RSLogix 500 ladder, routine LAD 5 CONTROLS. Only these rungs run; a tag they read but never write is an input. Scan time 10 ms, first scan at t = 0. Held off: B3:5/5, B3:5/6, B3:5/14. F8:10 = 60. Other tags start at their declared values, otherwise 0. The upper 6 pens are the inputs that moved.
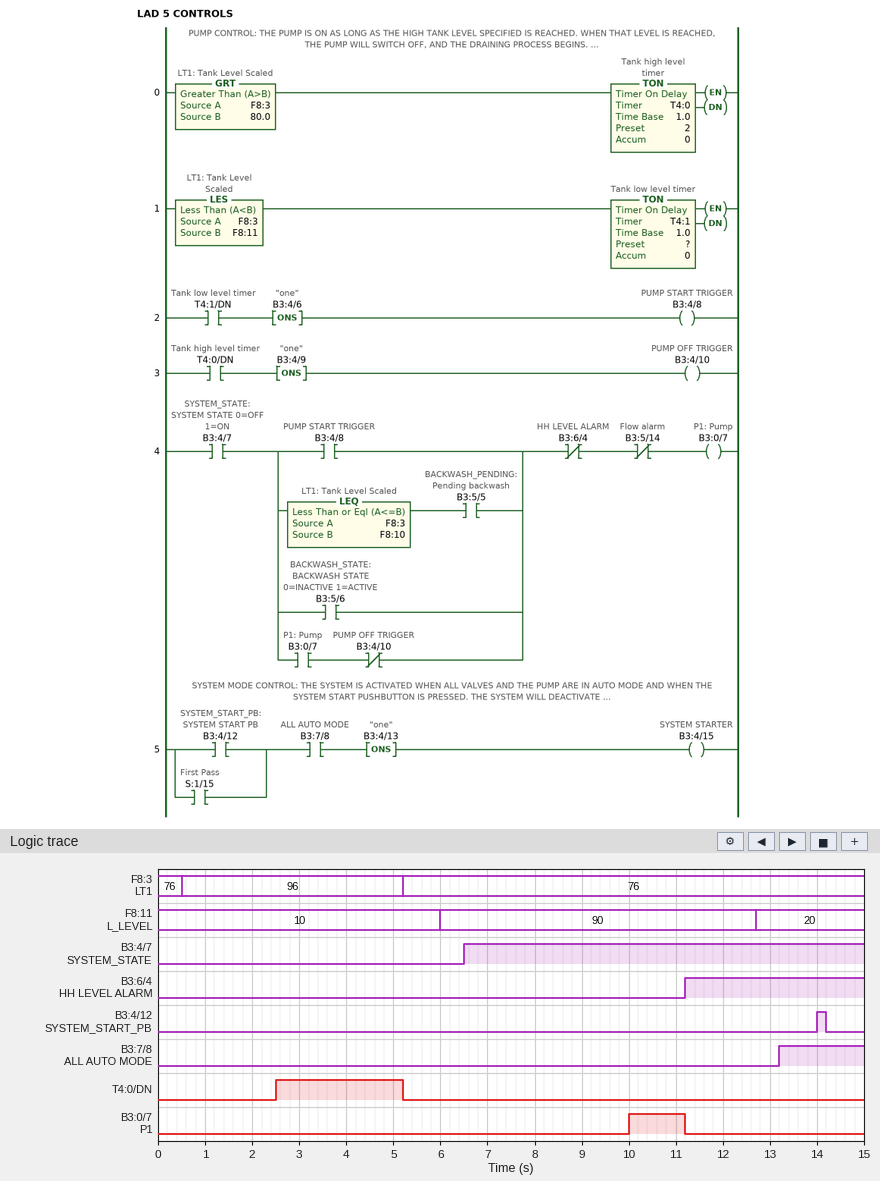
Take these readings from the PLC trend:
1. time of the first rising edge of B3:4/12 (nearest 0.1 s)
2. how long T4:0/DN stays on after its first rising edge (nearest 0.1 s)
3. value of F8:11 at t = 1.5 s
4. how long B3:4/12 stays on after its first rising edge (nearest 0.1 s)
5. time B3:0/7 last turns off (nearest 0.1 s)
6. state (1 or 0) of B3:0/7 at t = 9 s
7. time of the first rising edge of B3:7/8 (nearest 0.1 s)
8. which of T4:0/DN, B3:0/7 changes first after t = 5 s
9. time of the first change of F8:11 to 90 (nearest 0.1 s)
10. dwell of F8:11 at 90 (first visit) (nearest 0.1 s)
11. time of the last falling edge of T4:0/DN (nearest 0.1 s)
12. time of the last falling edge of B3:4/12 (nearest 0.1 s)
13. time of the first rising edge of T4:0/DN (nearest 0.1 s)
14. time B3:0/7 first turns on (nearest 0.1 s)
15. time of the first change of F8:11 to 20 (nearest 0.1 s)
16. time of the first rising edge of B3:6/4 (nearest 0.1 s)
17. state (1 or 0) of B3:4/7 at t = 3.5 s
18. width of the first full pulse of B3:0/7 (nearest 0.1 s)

14.0 s
2.7 s
10
0.2 s
11.2 s
0
13.2 s
T4:0/DN
6.0 s
6.7 s
5.2 s
14.2 s
2.5 s
10.0 s
12.7 s
11.2 s
0
1.2 s
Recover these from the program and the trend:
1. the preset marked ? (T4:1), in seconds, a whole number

4 s
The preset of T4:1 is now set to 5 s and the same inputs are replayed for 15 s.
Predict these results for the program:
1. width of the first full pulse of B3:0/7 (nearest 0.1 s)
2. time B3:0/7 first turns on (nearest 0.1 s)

0.2 s
11.0 s
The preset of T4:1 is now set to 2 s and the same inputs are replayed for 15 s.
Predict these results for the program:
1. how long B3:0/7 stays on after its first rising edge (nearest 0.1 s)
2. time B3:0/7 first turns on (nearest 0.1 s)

3.2 s
8.0 s
